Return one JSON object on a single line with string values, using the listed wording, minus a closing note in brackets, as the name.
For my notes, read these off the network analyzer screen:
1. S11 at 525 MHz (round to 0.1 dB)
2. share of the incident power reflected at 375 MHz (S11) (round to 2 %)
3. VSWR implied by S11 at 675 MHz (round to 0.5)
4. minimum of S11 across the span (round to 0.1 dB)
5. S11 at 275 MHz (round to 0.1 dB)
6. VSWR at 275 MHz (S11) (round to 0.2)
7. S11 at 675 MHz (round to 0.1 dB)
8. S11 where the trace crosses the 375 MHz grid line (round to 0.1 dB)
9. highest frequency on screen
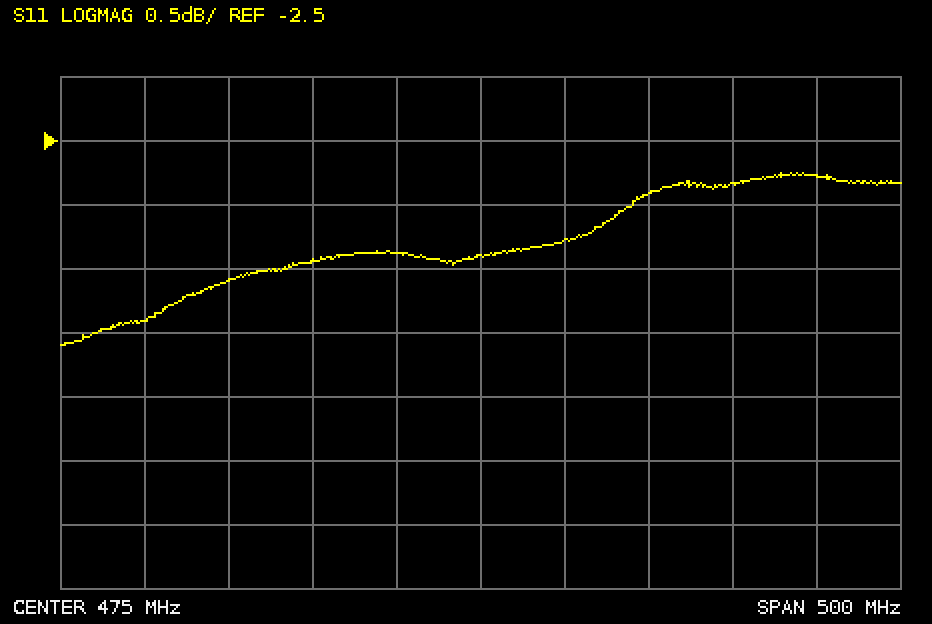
{"S11 at 525 MHz": "-3.3 dB", "share of the incident power reflected at 375 MHz (S11)": "46 %", "VSWR implied by S11 at 675 MHz": "6.5", "minimum of S11 across the span": "-4.1 dB", "S11 at 275 MHz": "-3.9 dB", "VSWR at 275 MHz (S11)": "4.6", "S11 at 675 MHz": "-2.8 dB", "S11 where the trace crosses the 375 MHz grid line": "-3.4 dB", "highest frequency on screen": "725 MHz"}
